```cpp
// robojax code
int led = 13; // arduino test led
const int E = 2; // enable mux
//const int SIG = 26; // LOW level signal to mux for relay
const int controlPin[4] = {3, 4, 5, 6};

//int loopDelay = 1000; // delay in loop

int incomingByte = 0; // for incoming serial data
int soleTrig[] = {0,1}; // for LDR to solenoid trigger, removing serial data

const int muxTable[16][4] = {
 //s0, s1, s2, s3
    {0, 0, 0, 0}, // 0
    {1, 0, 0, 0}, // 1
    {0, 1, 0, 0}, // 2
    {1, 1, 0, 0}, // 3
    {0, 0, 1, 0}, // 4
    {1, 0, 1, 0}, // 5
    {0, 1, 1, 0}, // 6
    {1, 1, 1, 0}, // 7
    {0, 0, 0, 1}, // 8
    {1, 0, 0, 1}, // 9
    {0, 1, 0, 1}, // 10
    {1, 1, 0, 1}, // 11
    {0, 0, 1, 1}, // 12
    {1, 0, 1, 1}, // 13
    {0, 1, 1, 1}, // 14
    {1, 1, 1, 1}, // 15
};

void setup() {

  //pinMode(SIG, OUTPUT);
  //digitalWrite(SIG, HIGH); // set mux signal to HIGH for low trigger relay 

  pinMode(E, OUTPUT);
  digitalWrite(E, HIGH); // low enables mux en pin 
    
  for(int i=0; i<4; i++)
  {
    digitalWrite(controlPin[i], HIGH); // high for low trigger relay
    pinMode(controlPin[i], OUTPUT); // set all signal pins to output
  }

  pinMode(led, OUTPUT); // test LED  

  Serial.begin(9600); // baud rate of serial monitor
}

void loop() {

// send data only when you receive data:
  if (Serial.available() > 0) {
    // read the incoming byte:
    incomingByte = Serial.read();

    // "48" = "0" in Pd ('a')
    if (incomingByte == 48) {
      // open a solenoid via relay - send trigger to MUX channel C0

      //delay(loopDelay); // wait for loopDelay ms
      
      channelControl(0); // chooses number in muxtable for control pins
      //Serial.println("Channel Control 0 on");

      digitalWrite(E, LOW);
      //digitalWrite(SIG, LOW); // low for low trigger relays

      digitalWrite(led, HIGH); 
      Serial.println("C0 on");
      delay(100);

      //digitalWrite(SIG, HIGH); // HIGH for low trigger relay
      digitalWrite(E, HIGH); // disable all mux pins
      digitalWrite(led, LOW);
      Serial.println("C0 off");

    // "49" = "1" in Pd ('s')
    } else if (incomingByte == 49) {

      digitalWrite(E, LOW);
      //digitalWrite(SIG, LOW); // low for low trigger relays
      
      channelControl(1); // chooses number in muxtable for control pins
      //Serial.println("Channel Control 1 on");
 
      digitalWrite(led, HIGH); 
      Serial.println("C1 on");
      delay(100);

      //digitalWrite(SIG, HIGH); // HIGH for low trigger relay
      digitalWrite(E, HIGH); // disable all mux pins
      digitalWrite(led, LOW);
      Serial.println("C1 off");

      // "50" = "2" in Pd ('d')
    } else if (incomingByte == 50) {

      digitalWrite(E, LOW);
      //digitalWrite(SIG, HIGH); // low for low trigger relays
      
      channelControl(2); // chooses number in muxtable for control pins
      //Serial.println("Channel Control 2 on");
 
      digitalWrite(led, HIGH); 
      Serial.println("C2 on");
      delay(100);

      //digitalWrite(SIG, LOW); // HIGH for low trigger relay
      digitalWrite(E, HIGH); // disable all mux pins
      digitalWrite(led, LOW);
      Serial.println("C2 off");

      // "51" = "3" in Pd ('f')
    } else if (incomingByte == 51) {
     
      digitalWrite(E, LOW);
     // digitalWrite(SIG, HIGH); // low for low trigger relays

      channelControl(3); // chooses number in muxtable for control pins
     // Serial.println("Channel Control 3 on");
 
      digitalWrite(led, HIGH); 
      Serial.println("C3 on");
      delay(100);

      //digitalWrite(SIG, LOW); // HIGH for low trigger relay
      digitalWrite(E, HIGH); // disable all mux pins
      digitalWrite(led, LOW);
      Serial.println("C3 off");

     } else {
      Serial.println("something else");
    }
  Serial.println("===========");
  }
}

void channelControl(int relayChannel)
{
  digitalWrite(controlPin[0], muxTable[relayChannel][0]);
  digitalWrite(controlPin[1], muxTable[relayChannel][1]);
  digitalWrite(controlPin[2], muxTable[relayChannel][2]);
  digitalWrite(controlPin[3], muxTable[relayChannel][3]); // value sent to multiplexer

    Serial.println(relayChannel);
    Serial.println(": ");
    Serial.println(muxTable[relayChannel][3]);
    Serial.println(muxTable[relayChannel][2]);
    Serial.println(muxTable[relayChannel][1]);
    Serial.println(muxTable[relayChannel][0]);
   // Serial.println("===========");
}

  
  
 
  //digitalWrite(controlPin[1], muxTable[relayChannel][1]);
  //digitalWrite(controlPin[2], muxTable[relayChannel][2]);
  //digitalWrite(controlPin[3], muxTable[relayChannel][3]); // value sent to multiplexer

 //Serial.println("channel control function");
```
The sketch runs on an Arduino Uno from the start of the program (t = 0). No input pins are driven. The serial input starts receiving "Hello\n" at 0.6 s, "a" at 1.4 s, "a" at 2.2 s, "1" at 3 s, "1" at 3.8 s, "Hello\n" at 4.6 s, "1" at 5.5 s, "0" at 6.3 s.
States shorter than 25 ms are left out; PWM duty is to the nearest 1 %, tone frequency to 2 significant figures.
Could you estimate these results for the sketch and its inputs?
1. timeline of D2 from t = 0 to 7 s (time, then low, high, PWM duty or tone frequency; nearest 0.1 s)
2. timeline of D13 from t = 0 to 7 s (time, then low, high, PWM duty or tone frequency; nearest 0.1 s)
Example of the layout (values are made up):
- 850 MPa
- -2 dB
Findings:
- 0 s high; 3 s low; 3.1 s high; 3.8 s low; 3.9 s high; 5.5 s low; 5.6 s high; 6.3 s low; 6.4 s high
- 0 s low; 3 s high; 3.1 s low; 3.8 s high; 3.9 s low; 5.5 s high; 5.6 s low; 6.3 s high; 6.4 s low
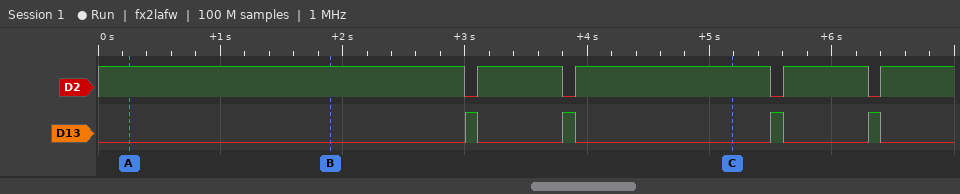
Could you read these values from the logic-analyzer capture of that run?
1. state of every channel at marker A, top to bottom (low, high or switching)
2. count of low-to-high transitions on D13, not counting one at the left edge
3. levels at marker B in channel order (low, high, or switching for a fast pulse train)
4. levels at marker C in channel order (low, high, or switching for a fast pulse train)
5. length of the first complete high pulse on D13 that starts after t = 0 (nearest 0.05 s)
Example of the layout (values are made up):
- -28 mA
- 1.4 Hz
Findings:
- D2 high, D13 low
- 4
- D2 high, D13 low
- D2 high, D13 low
- 0.10 s
